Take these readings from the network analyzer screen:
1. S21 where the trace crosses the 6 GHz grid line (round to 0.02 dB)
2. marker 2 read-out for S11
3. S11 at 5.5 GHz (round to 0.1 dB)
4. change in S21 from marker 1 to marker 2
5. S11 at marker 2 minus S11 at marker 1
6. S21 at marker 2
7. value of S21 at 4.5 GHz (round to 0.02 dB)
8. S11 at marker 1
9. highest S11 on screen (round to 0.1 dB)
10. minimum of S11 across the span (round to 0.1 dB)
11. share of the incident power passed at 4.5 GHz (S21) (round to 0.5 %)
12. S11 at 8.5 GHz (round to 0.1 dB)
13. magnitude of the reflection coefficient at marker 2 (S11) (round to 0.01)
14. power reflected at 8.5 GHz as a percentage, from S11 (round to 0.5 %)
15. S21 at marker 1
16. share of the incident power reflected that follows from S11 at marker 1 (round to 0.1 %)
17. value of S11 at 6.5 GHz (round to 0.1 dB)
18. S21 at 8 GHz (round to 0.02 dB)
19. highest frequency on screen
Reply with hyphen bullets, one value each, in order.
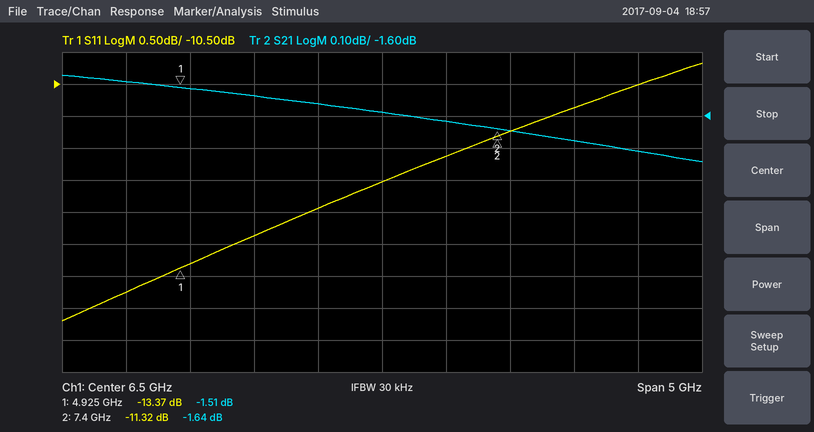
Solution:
- -1.56 dB
- -11.32 dB
- -12.9 dB
- -0.13 dB
- 2.05 dB
- -1.64 dB
- -1.50 dB
- -13.37 dB
- -10.2 dB
- -14.2 dB
- 71.0 %
- -10.5 dB
- 0.27
- 9.0 %
- -1.51 dB
- 4.6 %
- -12.0 dB
- -1.68 dB
- 9 GHz
